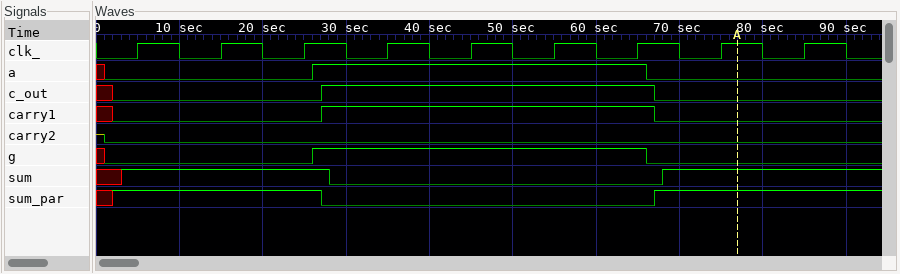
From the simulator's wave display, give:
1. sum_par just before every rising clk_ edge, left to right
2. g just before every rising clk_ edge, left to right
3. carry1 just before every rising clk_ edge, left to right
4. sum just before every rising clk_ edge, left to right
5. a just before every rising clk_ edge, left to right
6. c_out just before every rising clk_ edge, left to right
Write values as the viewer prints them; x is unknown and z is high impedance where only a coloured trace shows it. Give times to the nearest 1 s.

1 1 1 0 0 0 0 1 1
0 0 0 1 1 1 1 0 0
0 0 0 1 1 1 1 0 0
1 1 1 0 0 0 0 1 1
0 0 0 1 1 1 1 0 0
0 0 0 1 1 1 1 0 0
